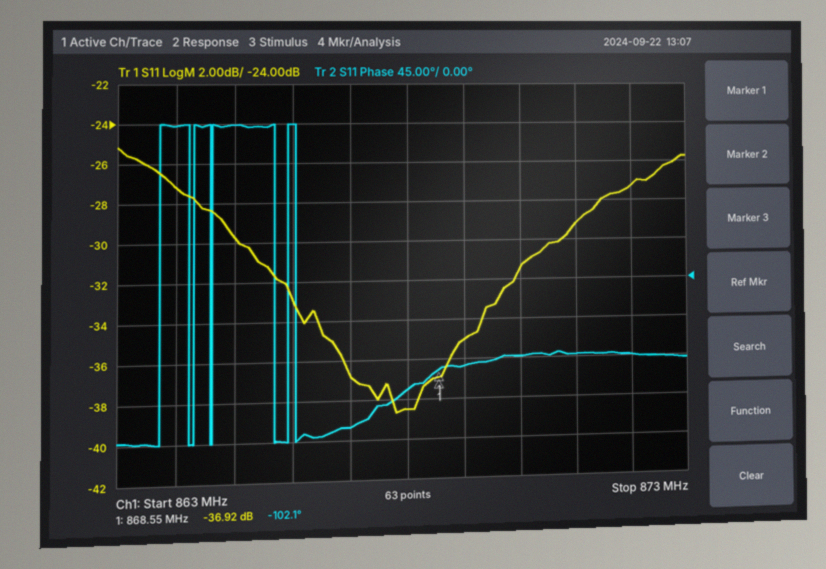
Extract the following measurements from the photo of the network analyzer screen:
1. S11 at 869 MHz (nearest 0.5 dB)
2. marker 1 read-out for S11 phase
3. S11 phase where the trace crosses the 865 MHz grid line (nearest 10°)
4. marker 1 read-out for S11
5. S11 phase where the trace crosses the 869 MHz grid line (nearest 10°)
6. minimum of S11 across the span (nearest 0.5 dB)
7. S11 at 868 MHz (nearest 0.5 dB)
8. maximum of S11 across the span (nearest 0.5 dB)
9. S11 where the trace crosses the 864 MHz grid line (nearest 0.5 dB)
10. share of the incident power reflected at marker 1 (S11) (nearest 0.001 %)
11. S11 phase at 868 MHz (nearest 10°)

-35.0 dB
-102.1°
180°
-36.92 dB
-100°
-38.5 dB
-38.5 dB
-25.0 dB
-27.0 dB
0.020 %
-120°
